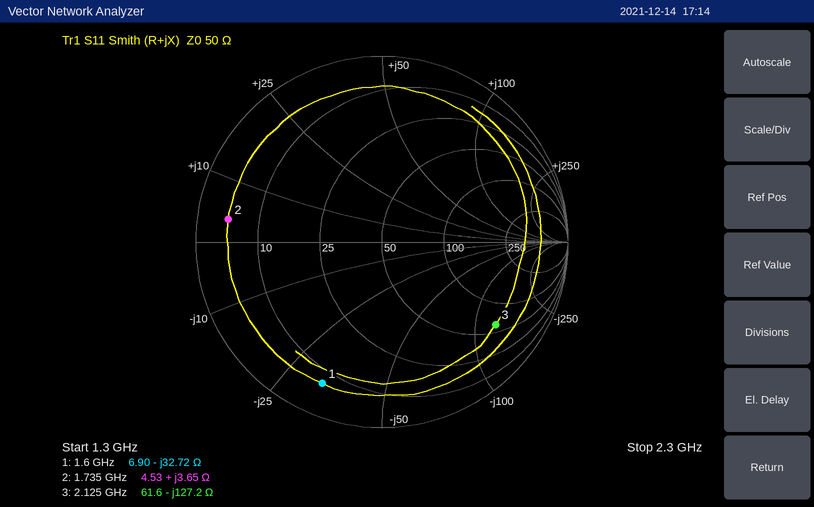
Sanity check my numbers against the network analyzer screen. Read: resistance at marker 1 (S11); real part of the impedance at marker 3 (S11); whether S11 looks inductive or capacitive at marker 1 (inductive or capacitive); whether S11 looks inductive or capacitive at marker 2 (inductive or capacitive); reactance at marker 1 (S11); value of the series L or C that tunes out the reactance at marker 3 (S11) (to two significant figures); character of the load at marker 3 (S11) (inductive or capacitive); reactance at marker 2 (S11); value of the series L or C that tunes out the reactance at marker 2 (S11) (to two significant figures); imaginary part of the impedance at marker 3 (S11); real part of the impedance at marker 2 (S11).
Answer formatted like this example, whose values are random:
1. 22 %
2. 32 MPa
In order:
1. 6.90 Ω
2. 61.6 Ω
3. capacitive
4. inductive
5. -32.72 Ω
6. 9.5 nH
7. capacitive
8. +3.65 Ω
9. 25 pF
10. -127.2 Ω
11. 4.53 Ω
